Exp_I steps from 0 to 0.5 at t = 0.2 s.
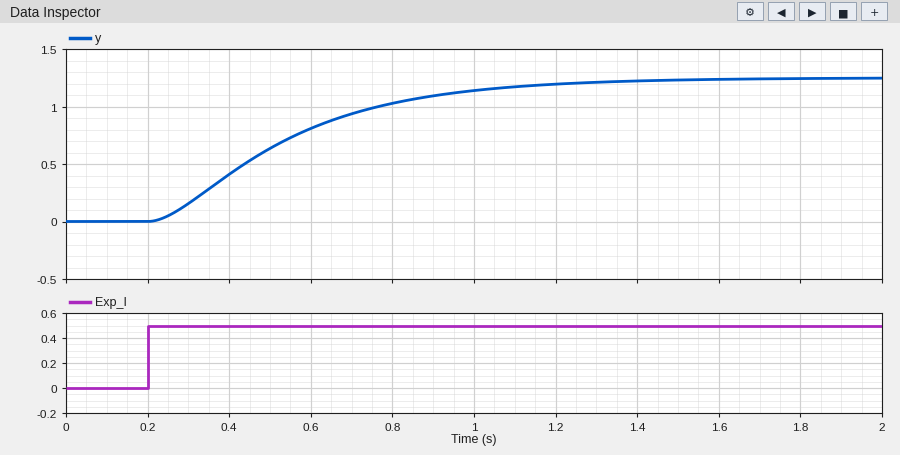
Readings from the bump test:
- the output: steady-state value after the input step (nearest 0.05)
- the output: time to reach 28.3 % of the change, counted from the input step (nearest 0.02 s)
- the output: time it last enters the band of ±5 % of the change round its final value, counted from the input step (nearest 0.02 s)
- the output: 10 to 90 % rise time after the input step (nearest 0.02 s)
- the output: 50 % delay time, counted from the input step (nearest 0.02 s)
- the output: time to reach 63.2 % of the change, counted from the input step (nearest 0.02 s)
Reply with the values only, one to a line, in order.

1.25
0.18 s
0.96 s
0.68 s
0.30 s
0.38 s
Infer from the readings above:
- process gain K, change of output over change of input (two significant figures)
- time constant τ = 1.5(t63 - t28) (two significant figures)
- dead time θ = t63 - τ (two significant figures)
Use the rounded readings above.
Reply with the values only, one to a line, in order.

2.5
0.30 s
0.080 s
